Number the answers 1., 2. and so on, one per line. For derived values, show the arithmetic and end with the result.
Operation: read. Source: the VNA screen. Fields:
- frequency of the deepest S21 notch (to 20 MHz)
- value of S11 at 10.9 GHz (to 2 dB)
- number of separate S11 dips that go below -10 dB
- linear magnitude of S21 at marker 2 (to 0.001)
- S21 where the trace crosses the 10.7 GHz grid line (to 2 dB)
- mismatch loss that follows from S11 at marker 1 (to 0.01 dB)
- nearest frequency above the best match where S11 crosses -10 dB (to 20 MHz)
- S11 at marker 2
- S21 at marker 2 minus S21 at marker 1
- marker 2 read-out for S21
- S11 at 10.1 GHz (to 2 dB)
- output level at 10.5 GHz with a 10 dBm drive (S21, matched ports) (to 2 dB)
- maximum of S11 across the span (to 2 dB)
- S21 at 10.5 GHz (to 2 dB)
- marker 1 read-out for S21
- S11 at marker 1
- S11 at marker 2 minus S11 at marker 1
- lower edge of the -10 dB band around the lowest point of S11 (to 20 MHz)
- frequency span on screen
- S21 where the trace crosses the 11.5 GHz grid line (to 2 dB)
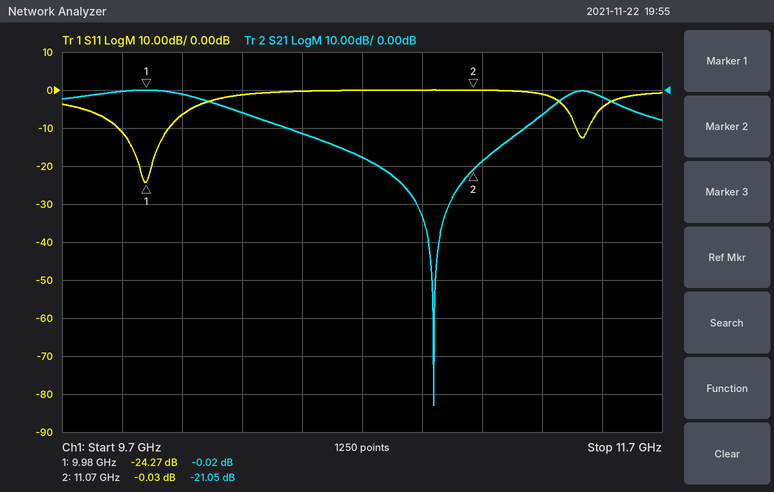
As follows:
1. 10.94 GHz
2. 0 dB
3. 2
4. 10^(-21.05/20) ≈ 0.089
5. -18 dB
6. −10 log10(1 − 10^(-24.27/10)) ≈ 0.02 dB
7. 10.06 GHz
8. -0.03 dB
9. -21.05 − (-0.02) = -21.03 dB
10. -21.05 dB
11. -6 dB
12. 10 dBm + (-12 dB) = -2 dBm
13. 0 dB
14. -12 dB
15. -0.02 dB
16. -24.27 dB
17. -0.03 − (-24.27) = 24.24 dB
18. 9.88 GHz
19. 2 GHz
20. -2 dB
